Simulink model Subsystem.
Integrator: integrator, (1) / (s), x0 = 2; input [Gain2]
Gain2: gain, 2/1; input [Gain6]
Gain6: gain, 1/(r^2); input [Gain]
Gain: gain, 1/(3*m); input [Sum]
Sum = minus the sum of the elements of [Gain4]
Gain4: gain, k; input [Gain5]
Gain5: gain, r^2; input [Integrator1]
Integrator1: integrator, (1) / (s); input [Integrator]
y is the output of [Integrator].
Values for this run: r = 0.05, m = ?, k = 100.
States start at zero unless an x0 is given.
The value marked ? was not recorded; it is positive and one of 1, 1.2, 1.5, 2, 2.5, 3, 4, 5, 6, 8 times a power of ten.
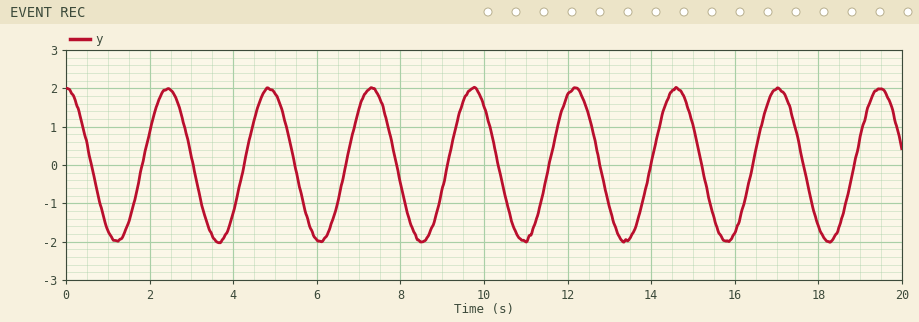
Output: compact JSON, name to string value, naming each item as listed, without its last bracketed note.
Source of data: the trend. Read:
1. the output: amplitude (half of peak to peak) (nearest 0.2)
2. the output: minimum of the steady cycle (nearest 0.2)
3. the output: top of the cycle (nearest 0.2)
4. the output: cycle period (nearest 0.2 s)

{"the output: amplitude (half of peak to peak)": "2.0", "the output: minimum of the steady cycle": "-2.0", "the output: top of the cycle": "2.0", "the output: cycle period": "2.4 s"}
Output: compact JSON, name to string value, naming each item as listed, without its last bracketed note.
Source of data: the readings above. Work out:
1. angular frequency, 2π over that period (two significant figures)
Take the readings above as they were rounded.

{"angular frequency, 2π over that period": "2.6 rad/s"}
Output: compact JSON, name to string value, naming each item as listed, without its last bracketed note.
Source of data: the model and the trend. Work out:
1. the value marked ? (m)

{"the value marked ?": "10"}
